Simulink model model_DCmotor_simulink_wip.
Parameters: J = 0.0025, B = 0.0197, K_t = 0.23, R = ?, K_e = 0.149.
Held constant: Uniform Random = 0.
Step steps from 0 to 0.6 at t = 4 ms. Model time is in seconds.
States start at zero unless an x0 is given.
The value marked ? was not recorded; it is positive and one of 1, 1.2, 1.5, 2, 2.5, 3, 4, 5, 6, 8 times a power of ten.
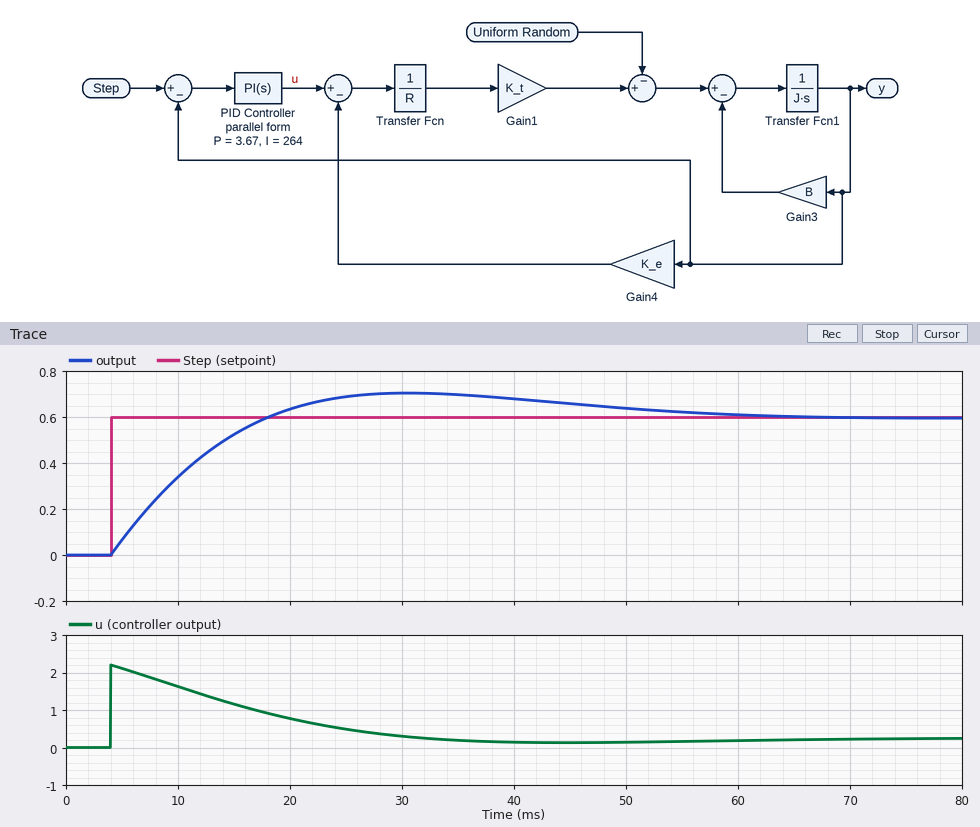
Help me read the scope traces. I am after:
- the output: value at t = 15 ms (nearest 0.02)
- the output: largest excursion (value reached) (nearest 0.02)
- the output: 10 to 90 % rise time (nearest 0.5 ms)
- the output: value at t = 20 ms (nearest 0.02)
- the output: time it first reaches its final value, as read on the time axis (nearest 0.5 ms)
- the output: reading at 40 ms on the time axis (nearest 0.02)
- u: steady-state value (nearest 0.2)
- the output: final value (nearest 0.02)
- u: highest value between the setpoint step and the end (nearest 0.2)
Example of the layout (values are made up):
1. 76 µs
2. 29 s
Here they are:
1. 0.52
2. 0.70
3. 10.5 ms
4. 0.64
5. 18.0 ms
6. 0.68
7. 0.2
8. 0.60
9. 2.2
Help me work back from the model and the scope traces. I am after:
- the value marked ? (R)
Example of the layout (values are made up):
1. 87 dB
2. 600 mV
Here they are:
1. 3
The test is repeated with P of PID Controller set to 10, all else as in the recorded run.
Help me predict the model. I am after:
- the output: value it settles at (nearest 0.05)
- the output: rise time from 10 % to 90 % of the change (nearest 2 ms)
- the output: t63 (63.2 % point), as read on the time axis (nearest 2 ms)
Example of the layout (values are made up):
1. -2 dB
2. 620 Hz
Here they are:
1. 0.60
2. 6 ms
3. 8 ms
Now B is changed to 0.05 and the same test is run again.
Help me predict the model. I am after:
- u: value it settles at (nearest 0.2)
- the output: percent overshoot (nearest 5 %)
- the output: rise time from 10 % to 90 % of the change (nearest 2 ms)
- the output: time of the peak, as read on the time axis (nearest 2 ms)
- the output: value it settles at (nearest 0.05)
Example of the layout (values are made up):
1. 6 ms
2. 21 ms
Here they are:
1. 0.4
2. 10 %
3. 12 ms
4. 32 ms
5. 0.60
